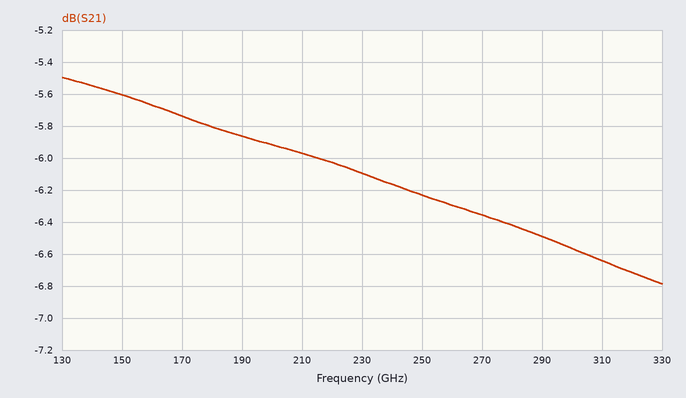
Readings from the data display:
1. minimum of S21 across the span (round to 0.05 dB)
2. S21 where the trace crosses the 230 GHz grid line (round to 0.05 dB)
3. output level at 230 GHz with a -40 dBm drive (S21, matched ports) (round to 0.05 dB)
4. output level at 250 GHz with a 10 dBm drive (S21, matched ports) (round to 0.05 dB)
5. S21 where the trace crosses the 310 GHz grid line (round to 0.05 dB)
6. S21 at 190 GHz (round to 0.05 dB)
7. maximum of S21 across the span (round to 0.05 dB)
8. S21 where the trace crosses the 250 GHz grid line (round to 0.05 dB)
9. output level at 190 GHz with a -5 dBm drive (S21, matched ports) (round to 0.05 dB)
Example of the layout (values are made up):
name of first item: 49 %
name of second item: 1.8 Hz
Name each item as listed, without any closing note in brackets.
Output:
minimum of S21 across the span: -6.80 dB
S21 where the trace crosses the 230 GHz grid line: -6.10 dB
output level at 230 GHz with a -40 dBm drive (S21, matched ports): -46.10 dBm
output level at 250 GHz with a 10 dBm drive (S21, matched ports): 3.75 dBm
S21 where the trace crosses the 310 GHz grid line: -6.65 dB
S21 at 190 GHz: -5.85 dB
maximum of S21 across the span: -5.50 dB
S21 where the trace crosses the 250 GHz grid line: -6.25 dB
output level at 190 GHz with a -5 dBm drive (S21, matched ports): -10.85 dBm
